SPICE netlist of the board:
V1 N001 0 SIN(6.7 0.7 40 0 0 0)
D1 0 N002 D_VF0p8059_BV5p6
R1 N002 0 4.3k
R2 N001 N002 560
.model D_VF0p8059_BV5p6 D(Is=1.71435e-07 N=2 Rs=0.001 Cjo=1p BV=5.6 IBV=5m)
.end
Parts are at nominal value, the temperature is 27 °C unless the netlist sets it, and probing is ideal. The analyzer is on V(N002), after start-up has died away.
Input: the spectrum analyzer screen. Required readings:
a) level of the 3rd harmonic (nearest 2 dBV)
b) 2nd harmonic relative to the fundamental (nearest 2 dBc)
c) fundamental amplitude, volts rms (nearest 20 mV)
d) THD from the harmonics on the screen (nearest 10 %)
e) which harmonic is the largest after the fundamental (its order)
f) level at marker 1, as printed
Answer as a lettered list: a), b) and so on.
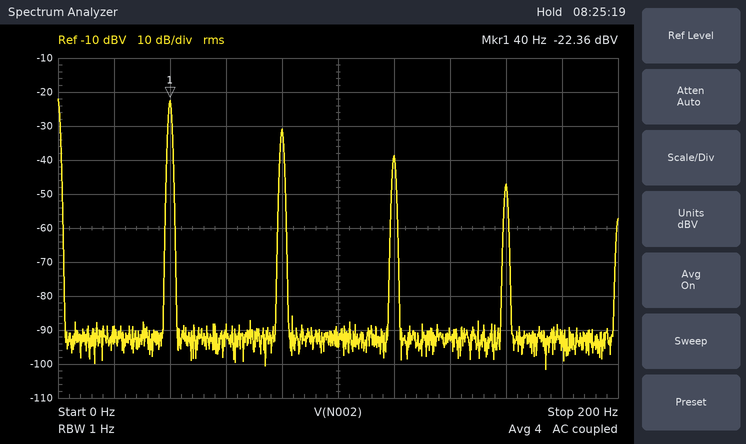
a) -38 dBV
b) -8 dBc
c) 80 mV
d) 40 %
e) 2
f) -22.36 dBV
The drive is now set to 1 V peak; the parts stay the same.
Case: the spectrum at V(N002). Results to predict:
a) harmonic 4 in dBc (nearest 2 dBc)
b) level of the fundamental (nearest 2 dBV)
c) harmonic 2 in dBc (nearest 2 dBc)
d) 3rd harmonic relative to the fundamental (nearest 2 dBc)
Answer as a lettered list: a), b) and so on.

a) -28 dBc
b) -16 dBV
c) -6 dBc
d) -14 dBc
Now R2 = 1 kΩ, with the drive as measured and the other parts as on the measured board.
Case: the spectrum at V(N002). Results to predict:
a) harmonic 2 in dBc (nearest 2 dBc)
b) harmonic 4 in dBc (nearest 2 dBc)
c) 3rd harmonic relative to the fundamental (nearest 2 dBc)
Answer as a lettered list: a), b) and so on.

a) -10 dBc
b) -28 dBc
c) -42 dBc
